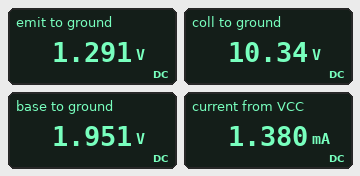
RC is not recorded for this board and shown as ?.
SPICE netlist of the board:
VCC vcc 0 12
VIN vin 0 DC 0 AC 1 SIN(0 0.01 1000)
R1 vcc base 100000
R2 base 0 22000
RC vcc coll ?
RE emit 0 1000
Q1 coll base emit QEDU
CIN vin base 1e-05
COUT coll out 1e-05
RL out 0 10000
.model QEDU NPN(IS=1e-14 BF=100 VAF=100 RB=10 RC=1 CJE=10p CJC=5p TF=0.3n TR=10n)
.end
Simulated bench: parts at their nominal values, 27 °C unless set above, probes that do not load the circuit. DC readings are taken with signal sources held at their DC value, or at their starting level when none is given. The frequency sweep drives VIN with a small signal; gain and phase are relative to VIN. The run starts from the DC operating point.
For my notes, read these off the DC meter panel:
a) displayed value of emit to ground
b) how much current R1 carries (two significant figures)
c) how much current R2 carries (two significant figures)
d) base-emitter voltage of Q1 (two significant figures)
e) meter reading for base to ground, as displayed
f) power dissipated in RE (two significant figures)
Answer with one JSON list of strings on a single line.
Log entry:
["1.291 V", "100 µA", "89 µA", "660 mV", "1.951 V", "1.7 mW"]
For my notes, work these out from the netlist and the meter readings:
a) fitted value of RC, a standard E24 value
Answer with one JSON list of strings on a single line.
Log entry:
["1.3 kΩ"]
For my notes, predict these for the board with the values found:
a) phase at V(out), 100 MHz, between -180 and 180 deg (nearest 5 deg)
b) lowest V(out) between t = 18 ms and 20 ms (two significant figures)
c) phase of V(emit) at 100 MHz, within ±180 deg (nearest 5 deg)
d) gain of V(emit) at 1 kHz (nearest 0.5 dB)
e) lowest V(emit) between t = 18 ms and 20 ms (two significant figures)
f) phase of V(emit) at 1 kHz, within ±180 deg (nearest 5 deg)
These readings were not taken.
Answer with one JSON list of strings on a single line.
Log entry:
["60 deg", "-11 mV", "0 deg", "0 dB", "1.3 V", "0 deg"]
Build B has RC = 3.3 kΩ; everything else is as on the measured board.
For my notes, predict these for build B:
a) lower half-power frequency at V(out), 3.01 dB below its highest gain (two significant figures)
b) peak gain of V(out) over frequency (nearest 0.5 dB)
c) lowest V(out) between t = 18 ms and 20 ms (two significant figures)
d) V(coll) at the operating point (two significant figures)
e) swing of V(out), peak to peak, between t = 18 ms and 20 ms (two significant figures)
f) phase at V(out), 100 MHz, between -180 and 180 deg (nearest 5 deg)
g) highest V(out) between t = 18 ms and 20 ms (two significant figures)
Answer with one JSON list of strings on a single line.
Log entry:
["1.7 Hz", "7.5 dB", "-24 mV", "7.8 V", "48 mV", "40 deg", "24 mV"]
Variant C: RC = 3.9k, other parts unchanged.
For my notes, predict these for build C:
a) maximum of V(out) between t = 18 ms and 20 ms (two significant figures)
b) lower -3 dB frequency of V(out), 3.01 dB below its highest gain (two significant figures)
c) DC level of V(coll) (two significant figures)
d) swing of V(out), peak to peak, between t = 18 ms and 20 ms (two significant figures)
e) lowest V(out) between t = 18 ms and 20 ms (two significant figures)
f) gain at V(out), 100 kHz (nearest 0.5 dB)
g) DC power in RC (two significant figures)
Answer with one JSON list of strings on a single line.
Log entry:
["27 mV", "1.7 Hz", "7.0 V", "54 mV", "-27 mV", "8.5 dB", "6.3 mW"]
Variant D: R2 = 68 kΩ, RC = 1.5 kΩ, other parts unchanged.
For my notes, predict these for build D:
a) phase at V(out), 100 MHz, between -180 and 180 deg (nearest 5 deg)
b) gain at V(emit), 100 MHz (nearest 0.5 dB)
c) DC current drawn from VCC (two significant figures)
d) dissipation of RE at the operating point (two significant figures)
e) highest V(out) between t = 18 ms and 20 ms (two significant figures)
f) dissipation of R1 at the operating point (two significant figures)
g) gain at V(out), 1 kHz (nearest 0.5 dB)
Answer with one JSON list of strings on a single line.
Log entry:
["50 deg", "0 dB", "3.1 mA", "9.1 mW", "13 mV", "690 µW", "2.0 dB"]
